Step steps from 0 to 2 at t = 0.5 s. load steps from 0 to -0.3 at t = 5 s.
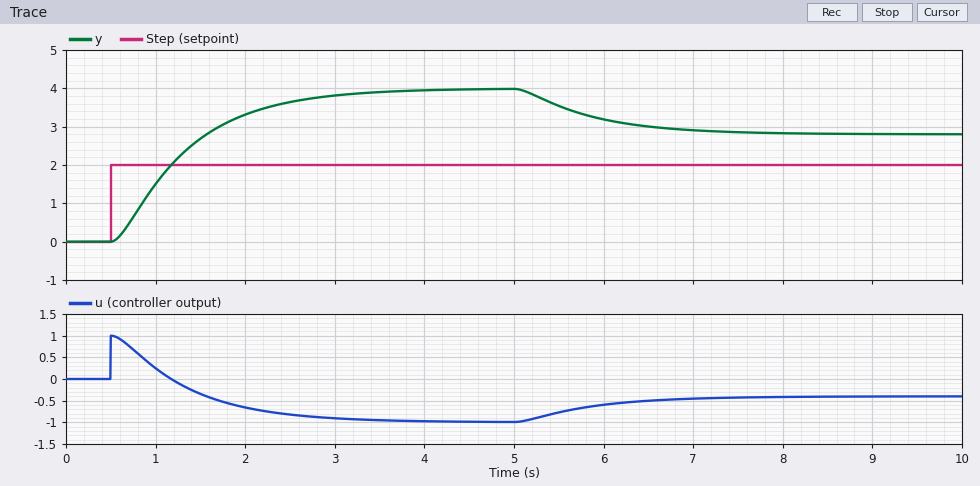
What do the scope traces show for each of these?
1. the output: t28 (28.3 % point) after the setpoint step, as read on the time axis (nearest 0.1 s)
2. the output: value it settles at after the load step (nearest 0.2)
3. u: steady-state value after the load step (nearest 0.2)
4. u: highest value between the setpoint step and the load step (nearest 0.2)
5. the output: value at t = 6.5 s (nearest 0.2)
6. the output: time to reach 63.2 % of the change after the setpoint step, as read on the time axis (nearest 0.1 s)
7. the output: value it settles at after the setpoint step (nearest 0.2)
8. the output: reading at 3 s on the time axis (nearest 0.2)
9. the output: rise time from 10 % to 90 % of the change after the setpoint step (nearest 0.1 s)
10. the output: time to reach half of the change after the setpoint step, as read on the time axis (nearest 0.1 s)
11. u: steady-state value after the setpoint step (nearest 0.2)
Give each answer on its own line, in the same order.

0.9 s
2.8
-0.4
1.0
3.0
1.4 s
4.0
3.8
1.7 s
1.2 s
-1.0
